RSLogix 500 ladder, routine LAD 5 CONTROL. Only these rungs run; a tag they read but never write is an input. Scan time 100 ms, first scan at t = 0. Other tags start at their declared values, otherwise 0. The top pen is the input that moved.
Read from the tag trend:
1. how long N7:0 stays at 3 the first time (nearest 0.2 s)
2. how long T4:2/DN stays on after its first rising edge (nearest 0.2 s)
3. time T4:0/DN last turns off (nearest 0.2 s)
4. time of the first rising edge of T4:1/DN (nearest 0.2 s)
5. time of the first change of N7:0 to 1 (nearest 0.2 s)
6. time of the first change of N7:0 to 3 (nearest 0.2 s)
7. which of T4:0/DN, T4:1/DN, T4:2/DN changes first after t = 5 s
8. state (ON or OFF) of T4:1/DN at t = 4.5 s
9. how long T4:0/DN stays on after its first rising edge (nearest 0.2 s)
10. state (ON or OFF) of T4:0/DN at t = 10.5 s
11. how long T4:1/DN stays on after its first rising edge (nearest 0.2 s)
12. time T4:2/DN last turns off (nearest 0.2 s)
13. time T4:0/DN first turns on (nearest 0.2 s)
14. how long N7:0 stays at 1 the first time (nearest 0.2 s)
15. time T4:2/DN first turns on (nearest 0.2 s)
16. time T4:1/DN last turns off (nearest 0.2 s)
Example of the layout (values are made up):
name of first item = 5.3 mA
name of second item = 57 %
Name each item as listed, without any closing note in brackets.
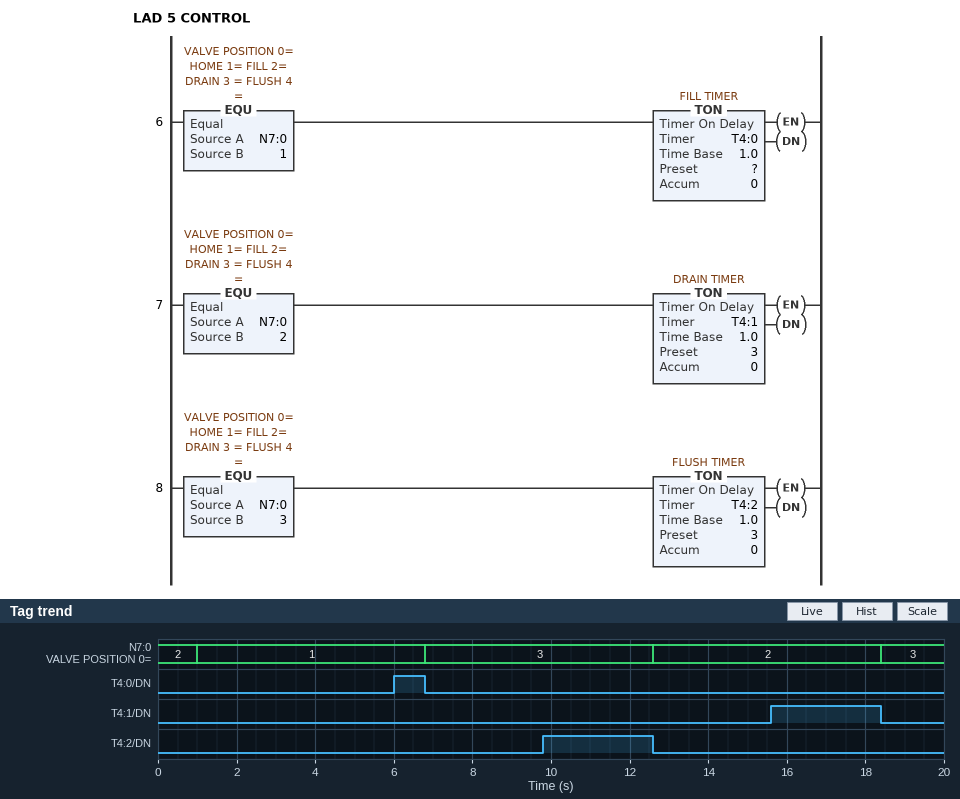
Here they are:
how long N7:0 stays at 3 the first time = 5.8 s
how long T4:2/DN stays on after its first rising edge = 2.8 s
time T4:0/DN last turns off = 6.8 s
time of the first rising edge of T4:1/DN = 15.6 s
time of the first change of N7:0 to 1 = 1.0 s
time of the first change of N7:0 to 3 = 6.8 s
which of T4:0/DN, T4:1/DN, T4:2/DN changes first after t = 5 s = T4:0/DN
state (ON or OFF) of T4:1/DN at t = 4.5 s = OFF
how long T4:0/DN stays on after its first rising edge = 0.8 s
state (ON or OFF) of T4:0/DN at t = 10.5 s = OFF
how long T4:1/DN stays on after its first rising edge = 2.8 s
time T4:2/DN last turns off = 12.6 s
time T4:0/DN first turns on = 6.0 s
how long N7:0 stays at 1 the first time = 5.8 s
time T4:2/DN first turns on = 9.8 s
time T4:1/DN last turns off = 18.4 s
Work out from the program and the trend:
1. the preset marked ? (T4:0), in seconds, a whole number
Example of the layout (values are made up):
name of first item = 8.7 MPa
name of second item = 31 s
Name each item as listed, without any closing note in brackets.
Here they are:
the preset marked ? (T4:0), in seconds, a whole number = 5 s
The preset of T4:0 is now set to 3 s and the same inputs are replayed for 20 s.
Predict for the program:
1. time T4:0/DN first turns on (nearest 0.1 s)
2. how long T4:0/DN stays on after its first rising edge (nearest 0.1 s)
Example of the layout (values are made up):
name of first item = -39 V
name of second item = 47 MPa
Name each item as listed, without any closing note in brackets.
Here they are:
time T4:0/DN first turns on = 4.0 s
how long T4:0/DN stays on after its first rising edge = 2.8 s
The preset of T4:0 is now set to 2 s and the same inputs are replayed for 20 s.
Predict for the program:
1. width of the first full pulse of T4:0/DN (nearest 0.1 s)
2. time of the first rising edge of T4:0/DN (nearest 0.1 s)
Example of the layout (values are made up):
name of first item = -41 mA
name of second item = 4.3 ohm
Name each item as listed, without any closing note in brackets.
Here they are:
width of the first full pulse of T4:0/DN = 3.8 s
time of the first rising edge of T4:0/DN = 3.0 s
